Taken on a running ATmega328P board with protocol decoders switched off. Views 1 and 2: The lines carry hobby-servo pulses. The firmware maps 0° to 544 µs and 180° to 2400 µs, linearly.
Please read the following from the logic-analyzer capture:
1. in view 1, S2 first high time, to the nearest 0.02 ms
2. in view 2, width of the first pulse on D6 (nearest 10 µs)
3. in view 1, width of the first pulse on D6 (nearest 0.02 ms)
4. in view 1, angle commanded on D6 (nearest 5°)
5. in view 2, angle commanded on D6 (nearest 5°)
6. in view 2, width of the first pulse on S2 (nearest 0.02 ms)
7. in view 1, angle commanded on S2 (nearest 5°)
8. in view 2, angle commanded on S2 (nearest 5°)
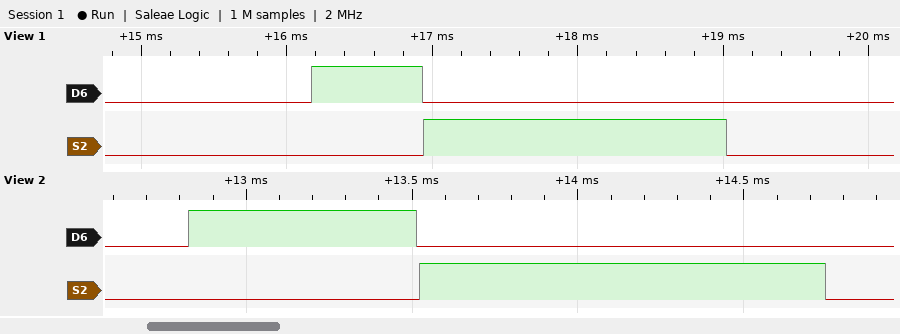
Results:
2.08 ms
690 µs
0.76 ms
20°
15°
1.22 ms
150°
65°
